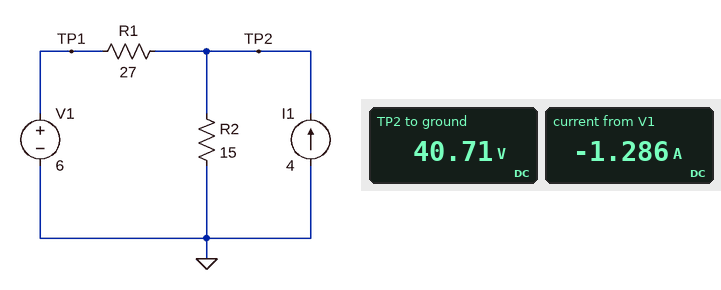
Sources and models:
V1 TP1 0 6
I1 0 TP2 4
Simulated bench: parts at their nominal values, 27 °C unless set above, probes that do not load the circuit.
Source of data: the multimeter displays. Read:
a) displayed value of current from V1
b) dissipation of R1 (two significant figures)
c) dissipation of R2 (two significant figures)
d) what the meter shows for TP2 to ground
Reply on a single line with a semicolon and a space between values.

-1.286 A; 45 W; 110 W; 40.71 V
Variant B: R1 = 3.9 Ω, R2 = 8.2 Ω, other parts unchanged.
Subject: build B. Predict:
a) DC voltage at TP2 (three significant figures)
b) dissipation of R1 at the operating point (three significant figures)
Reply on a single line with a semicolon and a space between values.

14.6 V; 19.1 W
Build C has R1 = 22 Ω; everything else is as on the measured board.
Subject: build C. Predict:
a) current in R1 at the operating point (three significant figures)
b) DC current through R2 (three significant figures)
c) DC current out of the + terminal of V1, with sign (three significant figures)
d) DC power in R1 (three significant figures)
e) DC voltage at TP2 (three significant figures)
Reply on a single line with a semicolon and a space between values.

1.46 A; 2.54 A; -1.46 A; 46.9 W; 38.1 V
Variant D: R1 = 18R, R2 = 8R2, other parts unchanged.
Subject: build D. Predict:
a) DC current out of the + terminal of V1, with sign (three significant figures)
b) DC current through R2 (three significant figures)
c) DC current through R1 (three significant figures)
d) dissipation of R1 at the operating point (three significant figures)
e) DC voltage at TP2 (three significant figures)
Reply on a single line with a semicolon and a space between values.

-1.02 A; 2.98 A; 1.02 A; 18.8 W; 24.4 V
